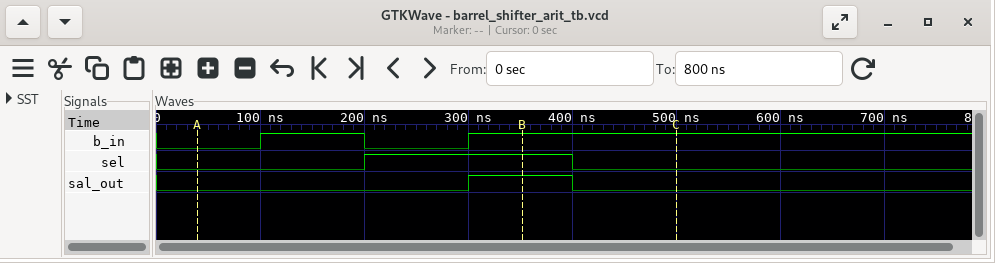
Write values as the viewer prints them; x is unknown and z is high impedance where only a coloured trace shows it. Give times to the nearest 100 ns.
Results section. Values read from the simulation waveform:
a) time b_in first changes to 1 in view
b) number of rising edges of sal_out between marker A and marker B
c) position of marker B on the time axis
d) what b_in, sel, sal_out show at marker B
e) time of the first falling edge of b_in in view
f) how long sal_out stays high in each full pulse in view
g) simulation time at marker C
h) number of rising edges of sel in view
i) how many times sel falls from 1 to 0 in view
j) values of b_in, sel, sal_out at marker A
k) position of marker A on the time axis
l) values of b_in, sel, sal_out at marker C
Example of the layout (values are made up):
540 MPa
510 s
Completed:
100 ns
1
400 ns
b_in=1, sel=1, sal_out=1
200 ns
100 ns
500 ns
1
1
b_in=0, sel=0, sal_out=0
0 ns
b_in=1, sel=0, sal_out=0
